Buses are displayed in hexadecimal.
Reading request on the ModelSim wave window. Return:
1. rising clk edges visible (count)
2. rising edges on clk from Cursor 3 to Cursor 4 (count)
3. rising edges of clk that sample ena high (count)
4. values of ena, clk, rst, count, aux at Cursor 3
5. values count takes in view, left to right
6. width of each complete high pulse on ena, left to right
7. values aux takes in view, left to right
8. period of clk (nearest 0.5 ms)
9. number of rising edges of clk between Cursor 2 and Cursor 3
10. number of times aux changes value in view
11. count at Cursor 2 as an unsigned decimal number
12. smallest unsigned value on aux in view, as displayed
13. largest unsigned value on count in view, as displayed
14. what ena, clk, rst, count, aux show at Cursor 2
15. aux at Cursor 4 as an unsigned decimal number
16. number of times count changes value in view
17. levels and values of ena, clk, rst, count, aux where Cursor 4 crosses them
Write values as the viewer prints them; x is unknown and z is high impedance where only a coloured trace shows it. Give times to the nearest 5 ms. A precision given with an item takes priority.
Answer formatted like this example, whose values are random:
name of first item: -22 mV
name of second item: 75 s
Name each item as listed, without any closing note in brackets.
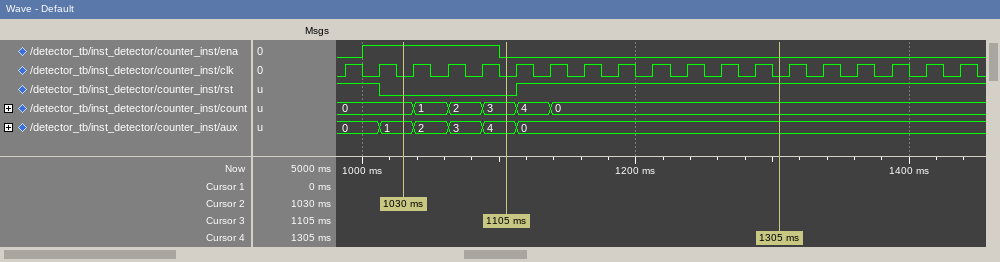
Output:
rising clk edges visible: 19
rising edges on clk from Cursor 3 to Cursor 4: 8
rising edges of clk that sample ena high: 4
values of ena, clk, rst, count, aux at Cursor 3: ena=0, clk=0, rst=0, count=3, aux=4
values count takes in view, left to right: 0, 1, 2, 3, 4, 0
width of each complete high pulse on ena, left to right: 100 ms
values aux takes in view, left to right: 0, 1, 2, 3, 4, 0
period of clk: 25 ms
number of rising edges of clk between Cursor 2 and Cursor 3: 3
number of times aux changes value in view: 5
count at Cursor 2 as an unsigned decimal number: 0
smallest unsigned value on aux in view, as displayed: 0
largest unsigned value on count in view, as displayed: 4
what ena, clk, rst, count, aux show at Cursor 2: ena=1, clk=0, rst=0, count=0, aux=1
aux at Cursor 4 as an unsigned decimal number: 0
number of times count changes value in view: 5
levels and values of ena, clk, rst, count, aux where Cursor 4 crosses them: ena=0, clk=0, rst=1, count=0, aux=0
